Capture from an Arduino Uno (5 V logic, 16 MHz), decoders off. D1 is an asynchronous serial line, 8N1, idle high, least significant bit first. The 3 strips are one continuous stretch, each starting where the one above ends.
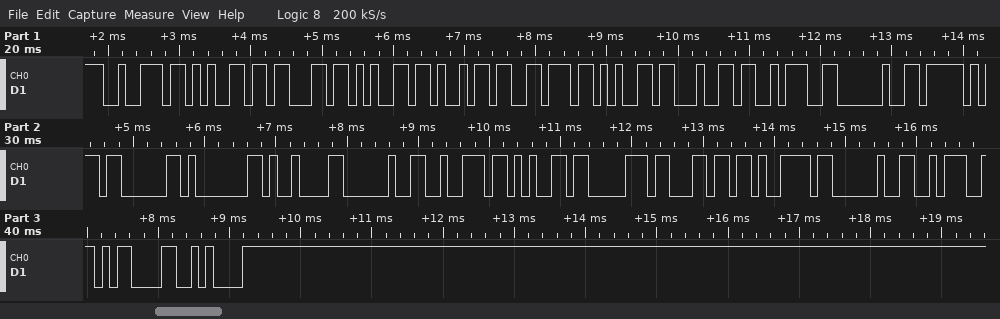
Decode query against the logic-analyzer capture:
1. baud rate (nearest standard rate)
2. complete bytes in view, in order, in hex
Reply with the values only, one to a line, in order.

9600 baud
0x72 0x65 0x63 0x65 0x69 0x76 0x65 0x64 0x3A 0x20 0x5F 0x03 0x01 0x09 0x20 0x72 0x65 0x70 0x6C 0x79 0x20 0x3A 0x0D 0x0A
